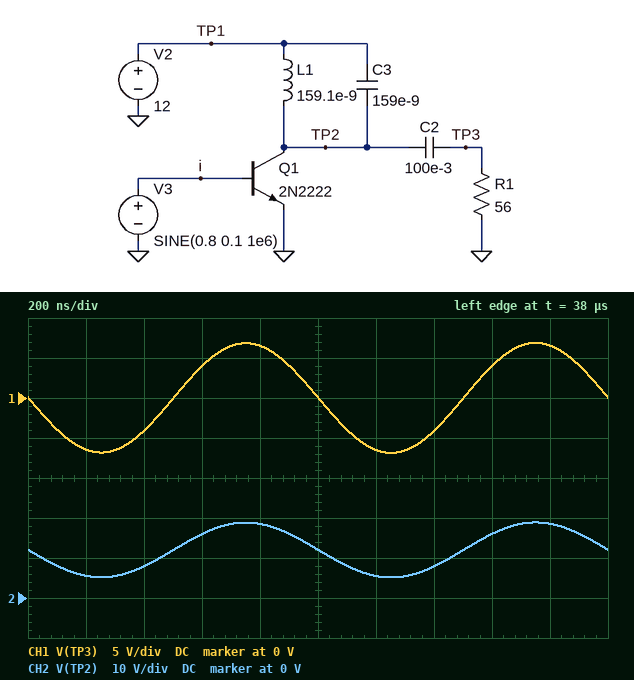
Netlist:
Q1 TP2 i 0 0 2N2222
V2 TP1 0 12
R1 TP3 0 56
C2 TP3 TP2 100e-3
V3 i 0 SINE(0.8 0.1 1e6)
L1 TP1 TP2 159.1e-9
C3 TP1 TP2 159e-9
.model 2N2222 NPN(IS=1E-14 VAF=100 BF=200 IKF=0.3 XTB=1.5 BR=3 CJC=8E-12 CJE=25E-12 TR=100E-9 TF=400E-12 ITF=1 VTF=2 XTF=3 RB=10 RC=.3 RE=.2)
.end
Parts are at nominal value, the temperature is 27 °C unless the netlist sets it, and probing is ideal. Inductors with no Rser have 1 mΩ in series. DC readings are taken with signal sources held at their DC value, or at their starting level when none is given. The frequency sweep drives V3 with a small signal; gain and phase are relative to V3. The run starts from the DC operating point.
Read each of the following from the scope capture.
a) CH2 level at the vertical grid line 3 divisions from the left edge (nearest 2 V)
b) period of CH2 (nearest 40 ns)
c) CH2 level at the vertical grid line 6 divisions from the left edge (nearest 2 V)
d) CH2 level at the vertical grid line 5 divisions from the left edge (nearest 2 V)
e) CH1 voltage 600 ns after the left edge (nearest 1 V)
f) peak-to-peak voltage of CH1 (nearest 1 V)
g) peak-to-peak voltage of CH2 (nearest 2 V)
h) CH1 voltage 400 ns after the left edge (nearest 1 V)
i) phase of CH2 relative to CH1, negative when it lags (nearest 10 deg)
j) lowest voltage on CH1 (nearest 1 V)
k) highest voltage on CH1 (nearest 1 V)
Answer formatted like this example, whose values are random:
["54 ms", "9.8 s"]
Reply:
["16 V", "1.00 µs", "6 V", "12 V", "4 V", "14 V", "14 V", "-4 V", "0 deg", "-7 V", "7 V"]
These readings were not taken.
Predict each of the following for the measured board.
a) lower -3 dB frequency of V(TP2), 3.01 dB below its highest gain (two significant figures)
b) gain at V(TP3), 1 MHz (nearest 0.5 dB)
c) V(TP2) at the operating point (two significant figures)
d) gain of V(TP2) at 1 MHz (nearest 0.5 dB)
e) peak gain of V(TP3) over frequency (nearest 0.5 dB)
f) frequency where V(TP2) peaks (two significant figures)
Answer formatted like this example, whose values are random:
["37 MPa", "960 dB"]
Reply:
["990 kHz", "38.5 dB", "12 V", "38.5 dB", "38.5 dB", "1.0 MHz"]
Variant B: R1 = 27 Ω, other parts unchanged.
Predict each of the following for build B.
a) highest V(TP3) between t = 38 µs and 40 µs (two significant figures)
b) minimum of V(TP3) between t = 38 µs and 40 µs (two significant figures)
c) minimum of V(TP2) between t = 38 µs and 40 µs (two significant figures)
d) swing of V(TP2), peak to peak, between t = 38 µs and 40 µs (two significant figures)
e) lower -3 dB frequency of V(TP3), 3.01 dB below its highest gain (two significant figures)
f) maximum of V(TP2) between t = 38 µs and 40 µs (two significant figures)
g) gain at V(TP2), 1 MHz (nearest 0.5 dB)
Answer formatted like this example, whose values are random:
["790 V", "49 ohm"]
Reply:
["3.8 V", "-3.8 V", "8.2 V", "7.6 V", "980 kHz", "16 V", "32.5 dB"]
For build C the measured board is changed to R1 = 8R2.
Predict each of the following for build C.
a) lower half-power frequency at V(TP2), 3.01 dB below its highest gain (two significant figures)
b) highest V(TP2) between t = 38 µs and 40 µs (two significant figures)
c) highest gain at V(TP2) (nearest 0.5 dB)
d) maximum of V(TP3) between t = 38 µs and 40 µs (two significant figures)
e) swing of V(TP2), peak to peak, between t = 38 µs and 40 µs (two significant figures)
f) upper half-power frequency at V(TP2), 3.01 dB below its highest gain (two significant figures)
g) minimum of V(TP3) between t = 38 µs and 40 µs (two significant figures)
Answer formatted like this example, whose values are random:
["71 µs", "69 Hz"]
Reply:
["940 kHz", "13 V", "22.5 dB", "1.2 V", "2.4 V", "1.1 MHz", "-1.2 V"]
